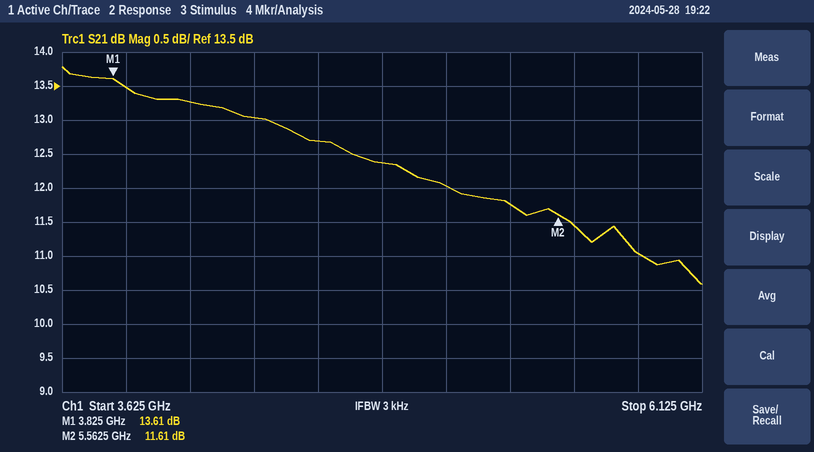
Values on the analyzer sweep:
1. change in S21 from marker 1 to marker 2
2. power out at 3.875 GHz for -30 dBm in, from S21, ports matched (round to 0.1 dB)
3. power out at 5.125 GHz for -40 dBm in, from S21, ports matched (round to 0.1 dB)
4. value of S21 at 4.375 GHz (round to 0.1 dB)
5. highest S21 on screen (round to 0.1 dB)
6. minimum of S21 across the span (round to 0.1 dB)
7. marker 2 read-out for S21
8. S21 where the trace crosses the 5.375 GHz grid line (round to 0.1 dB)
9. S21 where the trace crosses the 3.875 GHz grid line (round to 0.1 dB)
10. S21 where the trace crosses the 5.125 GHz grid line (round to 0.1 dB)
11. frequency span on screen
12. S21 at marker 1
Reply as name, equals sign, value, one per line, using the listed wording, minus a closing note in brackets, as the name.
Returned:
change in S21 from marker 1 to marker 2 = -2.00 dB
power out at 3.875 GHz for -30 dBm in, from S21, ports matched = -16.5 dBm
power out at 5.125 GHz for -40 dBm in, from S21, ports matched = -28.0 dBm
value of S21 at 4.375 GHz = 13.0 dB
highest S21 on screen = 13.8 dB
minimum of S21 across the span = 10.6 dB
marker 2 read-out for S21 = 11.61 dB
S21 where the trace crosses the 5.375 GHz grid line = 11.8 dB
S21 where the trace crosses the 3.875 GHz grid line = 13.5 dB
S21 where the trace crosses the 5.125 GHz grid line = 12.0 dB
frequency span on screen = 2.5 GHz
S21 at marker 1 = 13.61 dB
